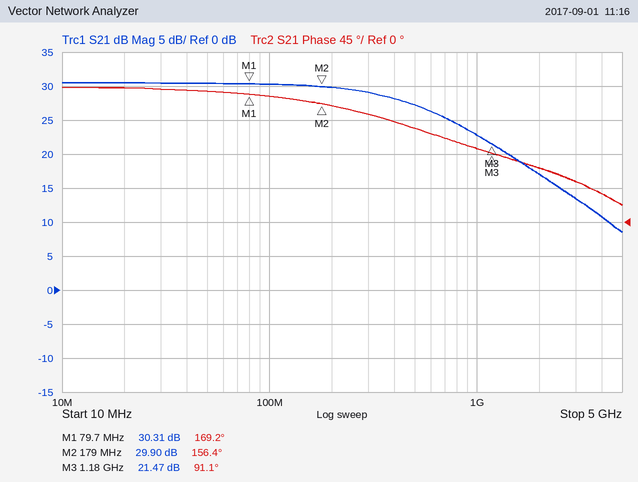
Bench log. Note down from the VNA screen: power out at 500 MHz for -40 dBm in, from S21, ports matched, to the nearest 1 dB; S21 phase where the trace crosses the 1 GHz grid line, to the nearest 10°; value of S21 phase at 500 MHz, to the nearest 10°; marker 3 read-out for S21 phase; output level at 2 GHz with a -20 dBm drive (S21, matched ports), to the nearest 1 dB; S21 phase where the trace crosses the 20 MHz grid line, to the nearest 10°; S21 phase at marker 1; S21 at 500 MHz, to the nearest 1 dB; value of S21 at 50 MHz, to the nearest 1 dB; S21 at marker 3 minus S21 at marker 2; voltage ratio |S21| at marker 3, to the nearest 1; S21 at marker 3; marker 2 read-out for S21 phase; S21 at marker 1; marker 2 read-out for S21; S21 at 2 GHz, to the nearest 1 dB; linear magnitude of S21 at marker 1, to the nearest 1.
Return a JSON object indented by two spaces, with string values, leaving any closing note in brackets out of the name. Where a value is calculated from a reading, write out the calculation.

{
  "power out at 500 MHz for -40 dBm in, from S21, ports matched, to the nearest 1 dB": "-40 dBm + (27 dB) = -13 dBm",
  "S21 phase where the trace crosses the 1 GHz grid line, to the nearest 10°": "100°",
  "value of S21 phase at 500 MHz, to the nearest 10°": "120°",
  "marker 3 read-out for S21 phase": "91.1°",
  "output level at 2 GHz with a -20 dBm drive (S21, matched ports), to the nearest 1 dB": "-20 dBm + (17 dB) = -3 dBm",
  "S21 phase where the trace crosses the 20 MHz grid line, to the nearest 10°": "180°",
  "S21 phase at marker 1": "169.2°",
  "S21 at 500 MHz, to the nearest 1 dB": "27 dB",
  "value of S21 at 50 MHz, to the nearest 1 dB": "30 dB",
  "S21 at marker 3 minus S21 at marker 2": "21.47 − (29.9) = -8.43 dB",
  "voltage ratio |S21| at marker 3, to the nearest 1": "10^(21.47/20) ≈ 12",
  "S21 at marker 3": "21.47 dB",
  "marker 2 read-out for S21 phase": "156.4°",
  "S21 at marker 1": "30.31 dB",
  "marker 2 read-out for S21": "29.90 dB",
  "S21 at 2 GHz, to the nearest 1 dB": "17 dB",
  "linear magnitude of S21 at marker 1, to the nearest 1": "10^(30.31/20) ≈ 33"
}
